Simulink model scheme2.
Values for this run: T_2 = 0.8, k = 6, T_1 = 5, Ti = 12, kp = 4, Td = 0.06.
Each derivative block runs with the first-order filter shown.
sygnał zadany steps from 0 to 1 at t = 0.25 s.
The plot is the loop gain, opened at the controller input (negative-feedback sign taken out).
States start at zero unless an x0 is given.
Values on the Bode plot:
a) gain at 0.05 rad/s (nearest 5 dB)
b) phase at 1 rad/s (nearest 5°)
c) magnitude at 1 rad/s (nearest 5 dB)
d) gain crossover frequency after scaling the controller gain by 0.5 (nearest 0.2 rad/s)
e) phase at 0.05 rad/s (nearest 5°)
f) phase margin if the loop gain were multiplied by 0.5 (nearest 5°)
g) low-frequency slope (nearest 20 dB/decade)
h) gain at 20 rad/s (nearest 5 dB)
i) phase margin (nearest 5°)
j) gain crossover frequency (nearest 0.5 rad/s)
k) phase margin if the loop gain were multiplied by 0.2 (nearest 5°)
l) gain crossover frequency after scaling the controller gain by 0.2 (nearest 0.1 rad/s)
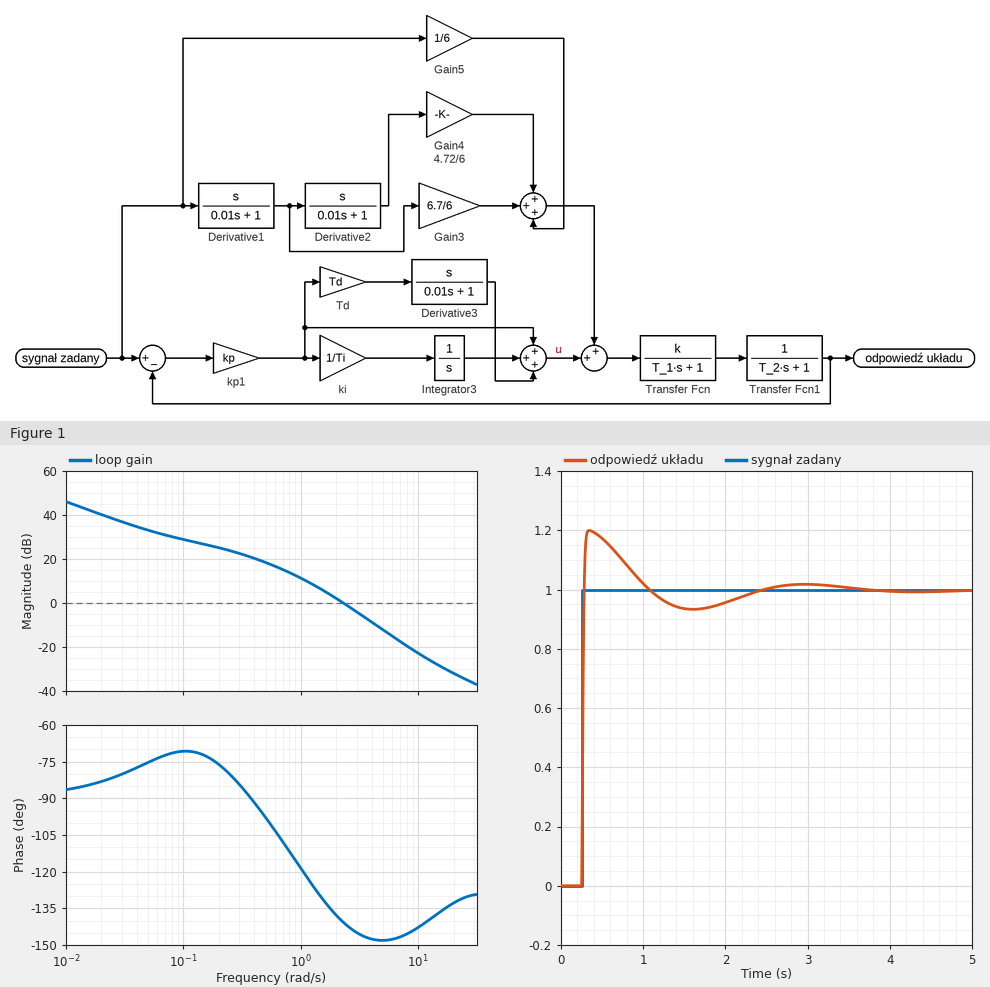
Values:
35 dB
-120°
10 dB
1.6 rad/s
-75°
50°
-20 dB/decade
-30 dB
40°
2.5 rad/s
70°
0.8 rad/s
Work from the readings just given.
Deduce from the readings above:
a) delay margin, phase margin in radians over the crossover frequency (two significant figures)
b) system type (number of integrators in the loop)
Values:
0.28 s
1
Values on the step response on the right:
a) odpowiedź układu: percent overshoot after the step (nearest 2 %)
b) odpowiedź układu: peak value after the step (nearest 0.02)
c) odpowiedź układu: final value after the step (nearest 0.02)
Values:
20 %
1.20
1.00
